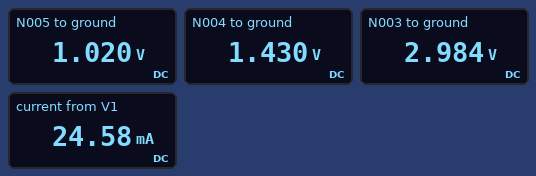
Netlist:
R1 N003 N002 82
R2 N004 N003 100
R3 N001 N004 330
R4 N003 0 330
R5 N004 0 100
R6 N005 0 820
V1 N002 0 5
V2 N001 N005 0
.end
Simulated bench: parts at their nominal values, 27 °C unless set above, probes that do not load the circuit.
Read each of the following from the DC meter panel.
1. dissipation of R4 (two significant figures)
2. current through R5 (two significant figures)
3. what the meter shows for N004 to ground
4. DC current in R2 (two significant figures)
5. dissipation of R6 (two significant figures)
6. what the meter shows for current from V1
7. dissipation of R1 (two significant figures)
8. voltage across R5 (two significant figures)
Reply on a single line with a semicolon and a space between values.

27 mW; 14 mA; 1.430 V; 16 mA; 1.3 mW; 24.58 mA; 50 mW; 1.4 V
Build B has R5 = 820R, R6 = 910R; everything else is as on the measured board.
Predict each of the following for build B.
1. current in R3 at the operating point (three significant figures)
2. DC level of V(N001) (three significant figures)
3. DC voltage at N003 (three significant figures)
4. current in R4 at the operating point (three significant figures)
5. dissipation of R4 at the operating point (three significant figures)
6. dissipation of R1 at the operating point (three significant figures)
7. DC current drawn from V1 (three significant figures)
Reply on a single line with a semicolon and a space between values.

2.42 mA; 2.20 V; 3.61 V; 10.9 mA; 39.4 mW; 23.7 mW; 17.0 mA
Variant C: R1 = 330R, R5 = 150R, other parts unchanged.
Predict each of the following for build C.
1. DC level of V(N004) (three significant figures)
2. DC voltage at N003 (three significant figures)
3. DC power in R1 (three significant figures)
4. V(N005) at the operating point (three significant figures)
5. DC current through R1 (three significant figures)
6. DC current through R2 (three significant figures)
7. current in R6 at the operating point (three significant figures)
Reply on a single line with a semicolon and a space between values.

834 mV; 1.46 V; 37.9 mW; 595 mV; 10.7 mA; 6.29 mA; 725 µA
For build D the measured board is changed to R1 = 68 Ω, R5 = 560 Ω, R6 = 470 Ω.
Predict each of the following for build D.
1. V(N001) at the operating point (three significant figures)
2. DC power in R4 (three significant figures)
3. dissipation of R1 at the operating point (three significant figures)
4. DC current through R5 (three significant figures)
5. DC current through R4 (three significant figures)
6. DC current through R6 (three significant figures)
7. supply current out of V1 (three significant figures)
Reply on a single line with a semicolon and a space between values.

1.65 V; 40.7 mW; 26.2 mW; 5.02 mA; 11.1 mA; 3.51 mA; 19.6 mA
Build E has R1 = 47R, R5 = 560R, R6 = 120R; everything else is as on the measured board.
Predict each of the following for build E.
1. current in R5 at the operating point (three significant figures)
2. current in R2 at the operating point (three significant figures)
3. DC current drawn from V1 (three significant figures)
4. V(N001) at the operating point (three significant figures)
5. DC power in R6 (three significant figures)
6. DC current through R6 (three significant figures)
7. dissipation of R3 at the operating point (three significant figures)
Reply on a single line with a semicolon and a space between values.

4.99 mA; 11.2 mA; 23.1 mA; 745 mV; 4.63 mW; 6.21 mA; 12.7 mW
